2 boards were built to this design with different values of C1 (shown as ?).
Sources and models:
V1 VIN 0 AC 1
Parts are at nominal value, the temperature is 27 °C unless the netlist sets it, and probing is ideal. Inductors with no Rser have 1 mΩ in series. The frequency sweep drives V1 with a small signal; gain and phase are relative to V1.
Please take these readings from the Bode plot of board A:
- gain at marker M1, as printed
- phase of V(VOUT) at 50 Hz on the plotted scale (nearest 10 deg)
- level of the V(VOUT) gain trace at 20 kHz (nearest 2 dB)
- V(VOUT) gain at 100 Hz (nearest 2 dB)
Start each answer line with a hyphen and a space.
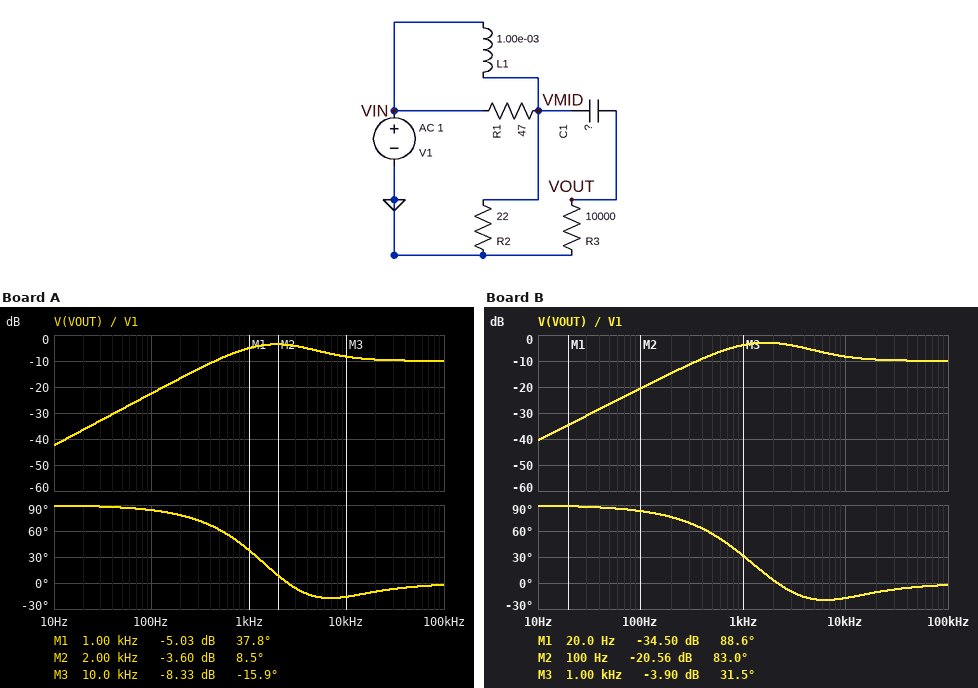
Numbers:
- -5.03 dB
- 90 deg
- -10 dB
- -22 dB
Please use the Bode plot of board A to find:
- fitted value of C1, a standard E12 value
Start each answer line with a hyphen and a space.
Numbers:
- 12 nF
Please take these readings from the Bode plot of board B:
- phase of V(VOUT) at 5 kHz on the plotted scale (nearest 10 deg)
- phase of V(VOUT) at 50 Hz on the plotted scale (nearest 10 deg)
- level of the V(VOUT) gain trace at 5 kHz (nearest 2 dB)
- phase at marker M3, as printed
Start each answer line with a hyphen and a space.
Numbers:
- -20 deg
- 90 deg
- -6 dB
- 31.5 deg
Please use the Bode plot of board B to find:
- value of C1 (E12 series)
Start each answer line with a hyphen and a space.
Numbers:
- 15 nF
